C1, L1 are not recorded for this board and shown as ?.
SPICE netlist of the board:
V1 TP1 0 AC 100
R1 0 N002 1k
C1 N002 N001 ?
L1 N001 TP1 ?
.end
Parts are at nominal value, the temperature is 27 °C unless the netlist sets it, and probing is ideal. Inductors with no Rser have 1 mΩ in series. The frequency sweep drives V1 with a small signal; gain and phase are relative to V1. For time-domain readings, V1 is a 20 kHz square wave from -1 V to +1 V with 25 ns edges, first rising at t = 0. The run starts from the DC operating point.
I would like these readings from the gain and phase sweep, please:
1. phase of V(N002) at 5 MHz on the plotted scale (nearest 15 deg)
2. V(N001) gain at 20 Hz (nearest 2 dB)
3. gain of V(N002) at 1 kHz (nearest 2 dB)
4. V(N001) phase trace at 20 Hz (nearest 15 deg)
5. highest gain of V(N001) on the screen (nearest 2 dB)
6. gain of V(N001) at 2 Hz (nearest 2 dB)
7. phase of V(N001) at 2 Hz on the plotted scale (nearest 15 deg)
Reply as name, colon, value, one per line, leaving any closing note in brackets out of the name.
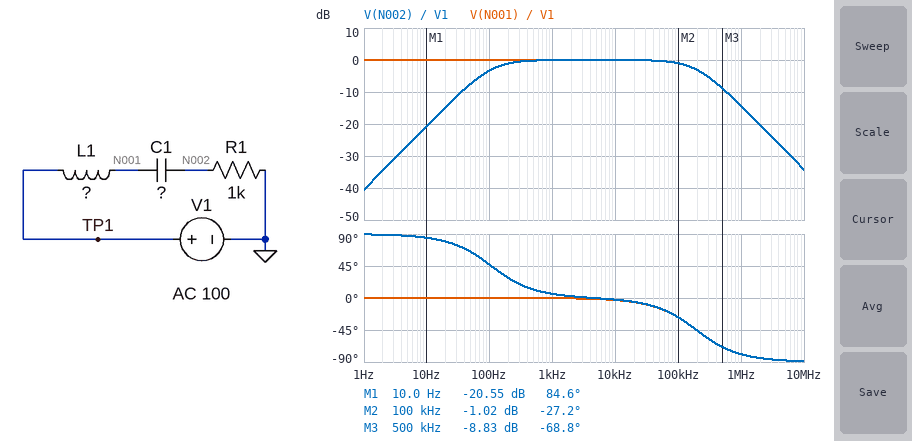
phase of V(N002) at 5 MHz on the plotted scale: -90 deg
V(N001) gain at 20 Hz: 0 dB
gain of V(N002) at 1 kHz: 0 dB
V(N001) phase trace at 20 Hz: 0 deg
highest gain of V(N001) on the screen: 0 dB
gain of V(N001) at 2 Hz: 0 dB
phase of V(N001) at 2 Hz on the plotted scale: 0 deg
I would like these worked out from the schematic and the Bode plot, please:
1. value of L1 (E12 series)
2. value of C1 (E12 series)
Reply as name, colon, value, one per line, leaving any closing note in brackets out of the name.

value of L1: 820 µH
value of C1: 1.5 µF
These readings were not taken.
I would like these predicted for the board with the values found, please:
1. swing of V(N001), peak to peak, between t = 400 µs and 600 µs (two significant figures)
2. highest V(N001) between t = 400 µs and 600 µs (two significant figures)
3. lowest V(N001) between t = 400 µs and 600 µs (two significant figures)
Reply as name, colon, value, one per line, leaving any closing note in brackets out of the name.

swing of V(N001), peak to peak, between t = 400 µs and 600 µs: 2.0 V
highest V(N001) between t = 400 µs and 600 µs: 1.0 V
lowest V(N001) between t = 400 µs and 600 µs: -1.0 V
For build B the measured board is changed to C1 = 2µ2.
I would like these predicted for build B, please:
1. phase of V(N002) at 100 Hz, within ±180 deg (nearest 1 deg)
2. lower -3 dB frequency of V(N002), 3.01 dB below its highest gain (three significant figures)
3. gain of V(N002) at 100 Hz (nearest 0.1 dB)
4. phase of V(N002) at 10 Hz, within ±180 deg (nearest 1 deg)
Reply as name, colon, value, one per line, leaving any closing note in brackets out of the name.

phase of V(N002) at 100 Hz, within ±180 deg: 36 deg
lower -3 dB frequency of V(N002), 3.01 dB below its highest gain: 72.3 Hz
gain of V(N002) at 100 Hz: -1.8 dB
phase of V(N002) at 10 Hz, within ±180 deg: 82 deg
